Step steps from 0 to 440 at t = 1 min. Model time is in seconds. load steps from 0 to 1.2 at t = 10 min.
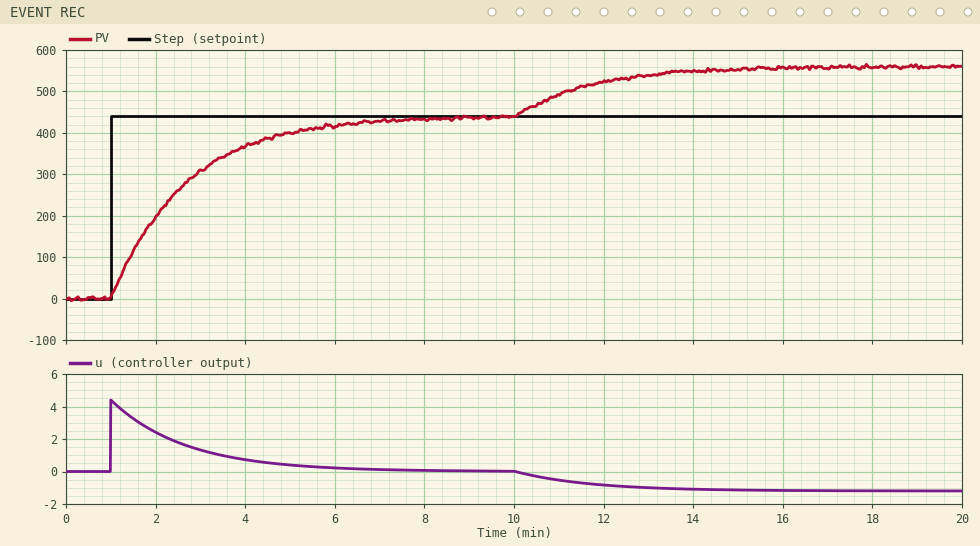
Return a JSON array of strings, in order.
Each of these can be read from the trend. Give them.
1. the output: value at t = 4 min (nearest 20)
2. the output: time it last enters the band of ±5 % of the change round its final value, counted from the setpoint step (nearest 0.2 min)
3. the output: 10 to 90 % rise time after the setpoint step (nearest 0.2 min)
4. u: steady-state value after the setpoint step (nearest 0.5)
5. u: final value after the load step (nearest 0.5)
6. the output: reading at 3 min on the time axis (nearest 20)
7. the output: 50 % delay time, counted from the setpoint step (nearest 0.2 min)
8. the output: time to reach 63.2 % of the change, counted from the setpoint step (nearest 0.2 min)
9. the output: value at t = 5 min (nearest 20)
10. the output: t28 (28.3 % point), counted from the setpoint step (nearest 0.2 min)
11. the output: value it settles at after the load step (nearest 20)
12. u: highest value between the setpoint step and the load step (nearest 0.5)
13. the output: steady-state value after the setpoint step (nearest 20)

["360", "5.0 min", "3.6 min", "0.0", "-1.0", "300", "1.2 min", "1.6 min", "400", "0.6 min", "560", "4.5", "440"]
